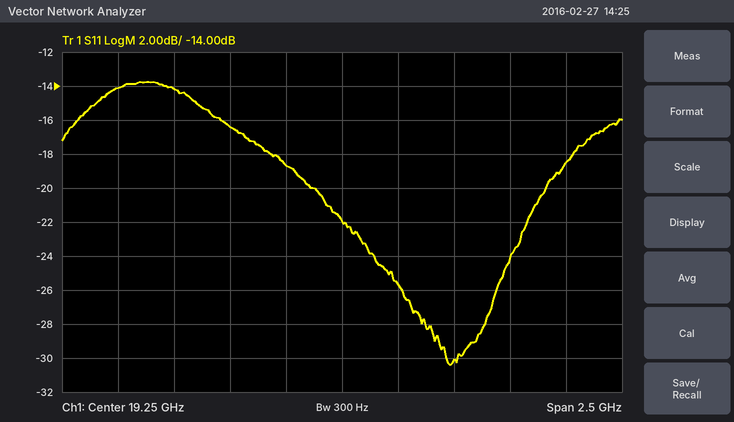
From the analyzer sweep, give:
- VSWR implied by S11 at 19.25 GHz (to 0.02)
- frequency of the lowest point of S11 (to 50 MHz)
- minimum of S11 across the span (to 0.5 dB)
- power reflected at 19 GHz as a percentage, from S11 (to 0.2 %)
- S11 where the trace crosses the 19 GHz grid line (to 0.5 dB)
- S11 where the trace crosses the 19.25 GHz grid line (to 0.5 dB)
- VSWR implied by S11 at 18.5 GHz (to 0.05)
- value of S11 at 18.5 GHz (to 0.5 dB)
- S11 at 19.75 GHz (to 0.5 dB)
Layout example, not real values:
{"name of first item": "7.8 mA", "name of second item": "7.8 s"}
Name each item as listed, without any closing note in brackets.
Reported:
{"VSWR implied by S11 at 19.25 GHz": "1.18", "frequency of the lowest point of S11": "19.75 GHz", "minimum of S11 across the span": "-30.5 dB", "power reflected at 19 GHz as a percentage, from S11": "1.4 %", "S11 where the trace crosses the 19 GHz grid line": "-18.5 dB", "S11 where the trace crosses the 19.25 GHz grid line": "-22.0 dB", "VSWR implied by S11 at 18.5 GHz": "1.50", "value of S11 at 18.5 GHz": "-14.0 dB", "S11 at 19.75 GHz": "-30.0 dB"}
